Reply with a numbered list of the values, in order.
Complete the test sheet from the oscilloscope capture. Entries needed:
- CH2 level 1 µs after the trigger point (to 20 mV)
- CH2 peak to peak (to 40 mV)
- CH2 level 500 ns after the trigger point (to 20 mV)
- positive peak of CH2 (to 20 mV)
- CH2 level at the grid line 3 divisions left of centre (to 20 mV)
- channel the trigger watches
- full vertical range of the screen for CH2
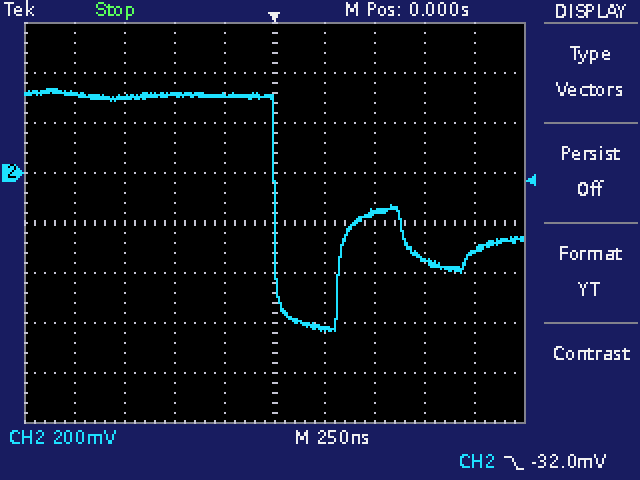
1. -320 mV
2. 960 mV
3. -160 mV
4. 340 mV
5. 300 mV
6. CH2
7. 1.6 V
